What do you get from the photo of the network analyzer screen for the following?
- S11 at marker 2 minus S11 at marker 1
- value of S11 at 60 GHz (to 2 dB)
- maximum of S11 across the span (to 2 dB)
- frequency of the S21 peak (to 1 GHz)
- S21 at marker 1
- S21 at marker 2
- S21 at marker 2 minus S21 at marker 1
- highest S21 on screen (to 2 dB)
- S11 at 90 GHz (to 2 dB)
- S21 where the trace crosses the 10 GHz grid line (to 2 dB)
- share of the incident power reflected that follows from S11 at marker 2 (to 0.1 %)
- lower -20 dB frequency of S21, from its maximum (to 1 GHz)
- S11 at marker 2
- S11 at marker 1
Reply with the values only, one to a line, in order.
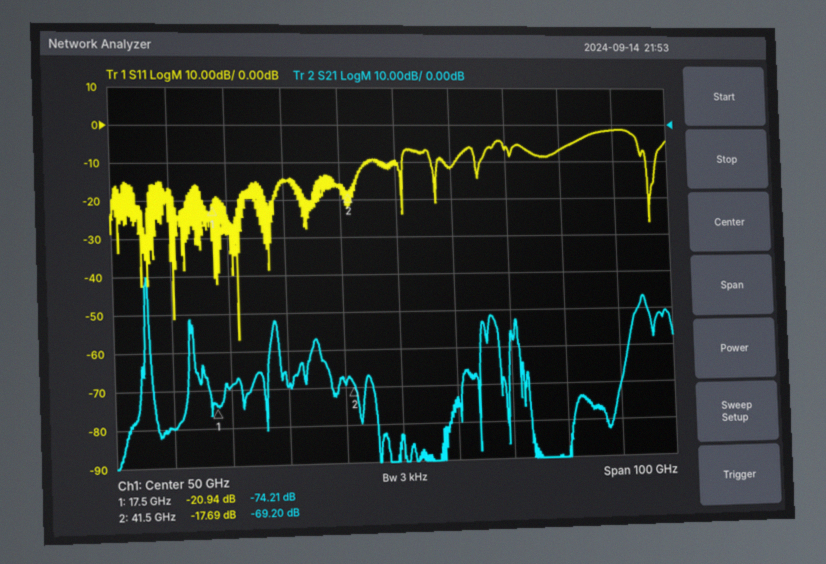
3.25 dB
-12 dB
-2 dB
6 GHz
-74.21 dB
-69.20 dB
5.01 dB
-40 dB
-2 dB
-80 dB
1.7 %
5 GHz
-17.69 dB
-20.94 dB
